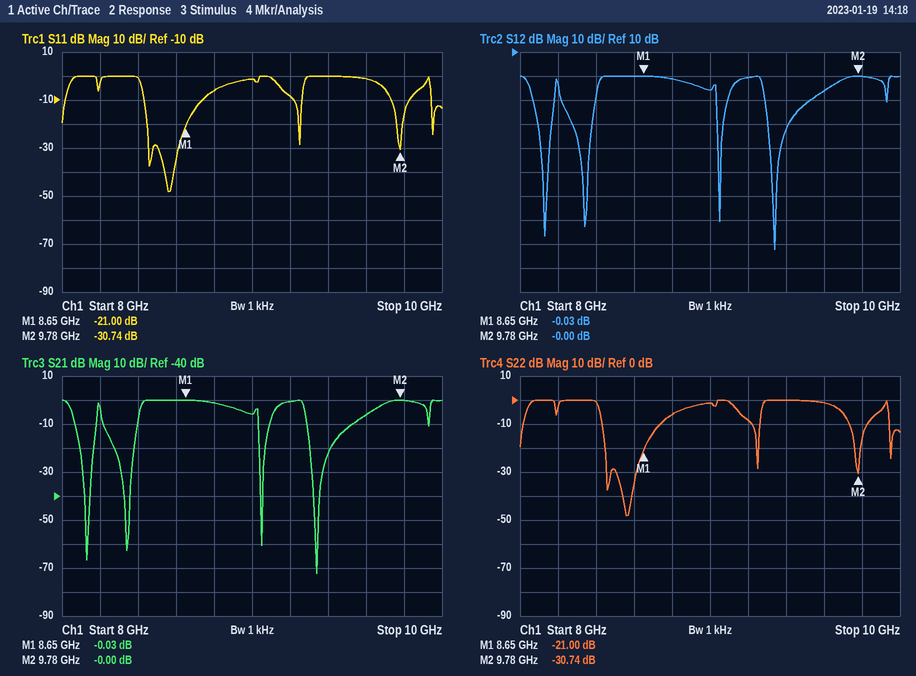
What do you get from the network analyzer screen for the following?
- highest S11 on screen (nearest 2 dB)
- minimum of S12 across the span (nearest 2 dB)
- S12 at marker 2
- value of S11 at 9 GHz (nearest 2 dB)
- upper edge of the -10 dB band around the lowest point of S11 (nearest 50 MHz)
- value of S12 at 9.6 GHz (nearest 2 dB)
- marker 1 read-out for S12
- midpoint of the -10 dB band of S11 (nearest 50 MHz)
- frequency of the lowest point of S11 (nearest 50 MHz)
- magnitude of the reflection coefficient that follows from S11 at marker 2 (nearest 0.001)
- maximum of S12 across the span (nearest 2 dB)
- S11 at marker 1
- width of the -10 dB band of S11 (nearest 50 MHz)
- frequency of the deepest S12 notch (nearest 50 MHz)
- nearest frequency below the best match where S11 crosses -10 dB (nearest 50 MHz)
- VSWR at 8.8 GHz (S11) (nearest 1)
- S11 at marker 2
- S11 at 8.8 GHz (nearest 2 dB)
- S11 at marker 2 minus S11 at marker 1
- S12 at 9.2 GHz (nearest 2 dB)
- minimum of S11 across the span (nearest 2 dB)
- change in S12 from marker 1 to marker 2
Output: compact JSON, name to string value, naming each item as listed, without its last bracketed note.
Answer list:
{"highest S11 on screen": "0 dB", "minimum of S12 across the span": "-72 dB", "S12 at marker 2": "-0.00 dB", "value of S11 at 9 GHz": "-2 dB", "upper edge of the -10 dB band around the lowest point of S11": "8.75 GHz", "value of S12 at 9.6 GHz": "-6 dB", "marker 1 read-out for S12": "-0.03 dB", "midpoint of the -10 dB band of S11": "8.60 GHz", "frequency of the lowest point of S11": "8.55 GHz", "magnitude of the reflection coefficient that follows from S11 at marker 2": "0.029", "maximum of S12 across the span": "0 dB", "S11 at marker 1": "-21.00 dB", "width of the -10 dB band of S11": "300 MHz", "frequency of the deepest S12 notch": "9.35 GHz", "nearest frequency below the best match where S11 crosses -10 dB": "8.45 GHz", "VSWR at 8.8 GHz (S11)": "3", "S11 at marker 2": "-30.74 dB", "S11 at 8.8 GHz": "-6 dB", "S11 at marker 2 minus S11 at marker 1": "-9.74 dB", "S12 at 9.2 GHz": "0 dB", "minimum of S11 across the span": "-48 dB", "change in S12 from marker 1 to marker 2": "0.03 dB"}
